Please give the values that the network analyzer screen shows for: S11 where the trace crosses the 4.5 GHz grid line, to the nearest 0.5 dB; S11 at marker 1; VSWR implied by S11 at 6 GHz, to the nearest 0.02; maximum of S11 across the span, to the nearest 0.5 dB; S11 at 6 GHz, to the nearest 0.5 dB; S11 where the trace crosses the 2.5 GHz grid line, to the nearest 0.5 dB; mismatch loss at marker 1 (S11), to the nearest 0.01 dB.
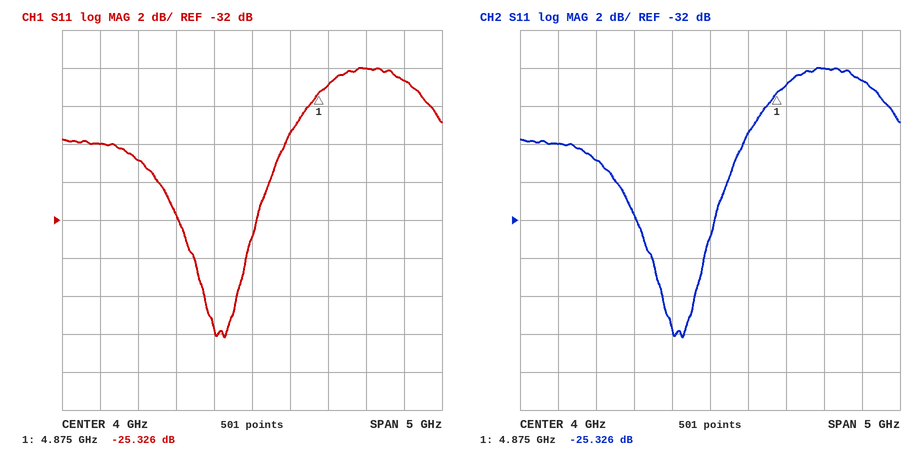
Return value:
-27.5 dB
-25.326 dB
1.12
-24.0 dB
-24.5 dB
-29.0 dB
0.01 dB
